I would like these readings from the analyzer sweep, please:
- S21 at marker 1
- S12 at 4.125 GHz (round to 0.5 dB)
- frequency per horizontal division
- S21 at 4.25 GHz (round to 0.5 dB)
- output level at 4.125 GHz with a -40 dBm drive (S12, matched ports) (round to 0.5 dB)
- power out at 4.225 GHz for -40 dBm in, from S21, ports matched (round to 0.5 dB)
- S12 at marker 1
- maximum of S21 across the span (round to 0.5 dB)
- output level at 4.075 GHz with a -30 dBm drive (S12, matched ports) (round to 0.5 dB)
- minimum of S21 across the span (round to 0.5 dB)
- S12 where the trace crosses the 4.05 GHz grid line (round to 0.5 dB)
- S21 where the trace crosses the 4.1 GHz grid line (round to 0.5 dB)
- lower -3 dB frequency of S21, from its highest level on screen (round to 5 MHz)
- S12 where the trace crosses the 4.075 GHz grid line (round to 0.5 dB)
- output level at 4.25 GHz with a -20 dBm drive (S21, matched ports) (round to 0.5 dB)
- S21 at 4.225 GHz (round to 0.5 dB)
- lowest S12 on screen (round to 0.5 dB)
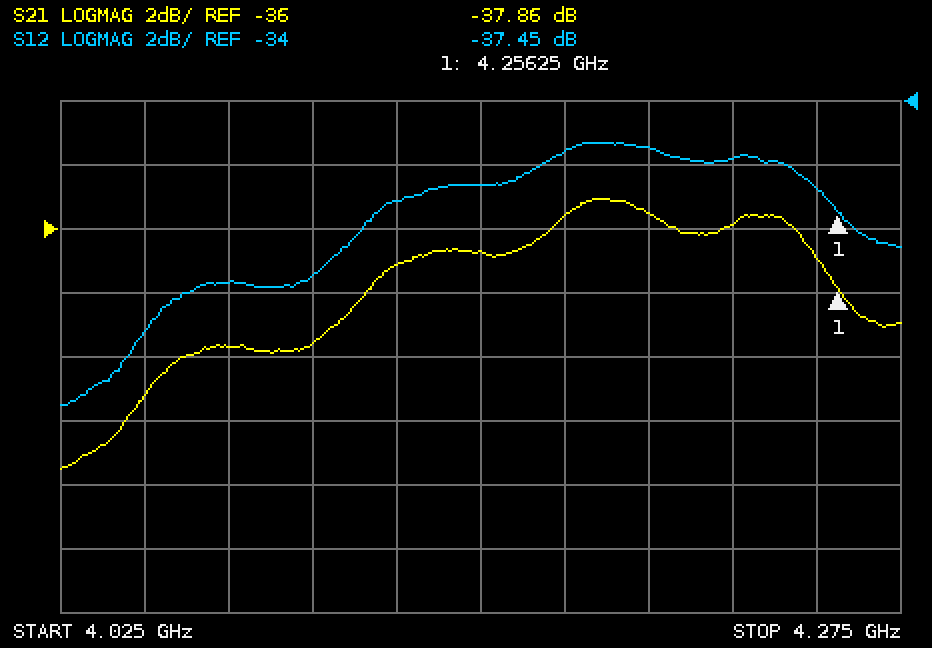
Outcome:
-37.86 dB
-37.0 dB
25 MHz
-37.0 dB
-77.0 dBm
-76.0 dBm
-37.45 dB
-35.0 dB
-69.5 dBm
-43.5 dB
-41.0 dB
-39.5 dB
4.115 GHz
-39.5 dB
-57.0 dBm
-36.0 dB
-43.5 dB
